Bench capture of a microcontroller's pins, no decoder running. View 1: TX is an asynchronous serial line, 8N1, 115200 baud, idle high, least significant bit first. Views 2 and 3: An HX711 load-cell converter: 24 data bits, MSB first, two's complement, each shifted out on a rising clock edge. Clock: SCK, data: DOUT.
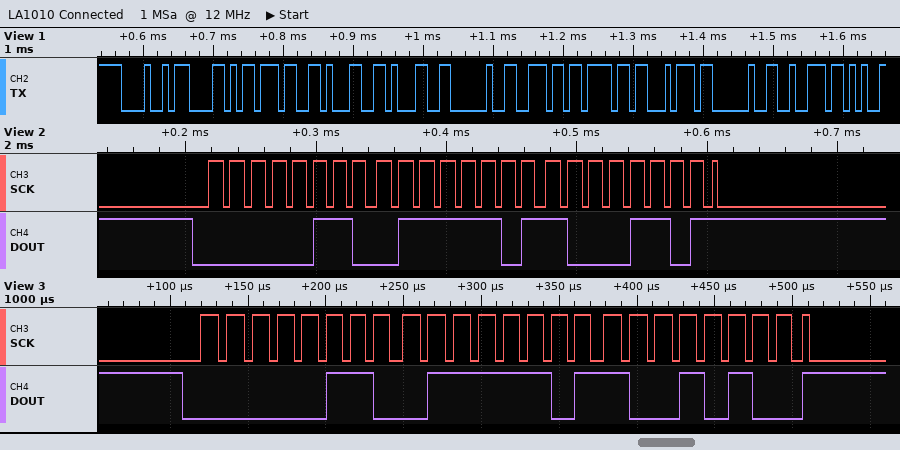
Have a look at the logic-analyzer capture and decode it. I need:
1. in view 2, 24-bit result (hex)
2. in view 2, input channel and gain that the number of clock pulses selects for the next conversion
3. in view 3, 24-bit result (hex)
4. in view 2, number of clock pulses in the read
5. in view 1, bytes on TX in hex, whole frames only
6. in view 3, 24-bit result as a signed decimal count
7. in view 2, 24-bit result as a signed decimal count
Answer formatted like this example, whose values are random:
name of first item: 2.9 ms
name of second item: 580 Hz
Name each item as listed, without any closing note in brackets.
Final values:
in view 2, 24-bit result: 0x067D8D
in view 2, input channel and gain that the number of clock pulses selects for the next conversion: channel A, gain 128
in view 3, 24-bit result: 0x067D94
in view 2, number of clock pulses in the read: 25
in view 1, bytes on TX in hex, whole frames only: 48 58 37 31 31 20 6E 6F 74 20 72
in view 3, 24-bit result as a signed decimal count: 425364
in view 2, 24-bit result as a signed decimal count: 425357
